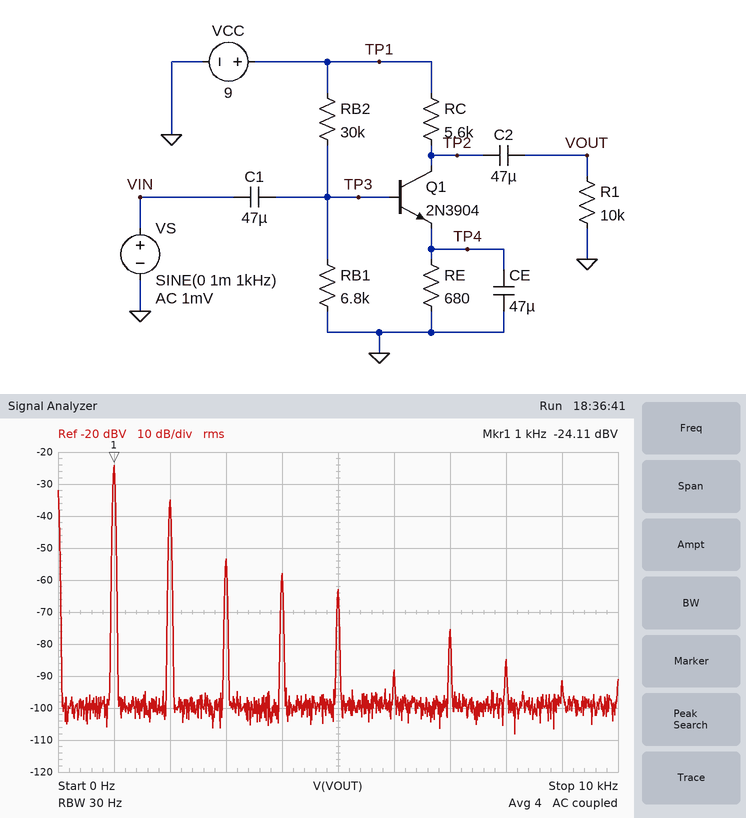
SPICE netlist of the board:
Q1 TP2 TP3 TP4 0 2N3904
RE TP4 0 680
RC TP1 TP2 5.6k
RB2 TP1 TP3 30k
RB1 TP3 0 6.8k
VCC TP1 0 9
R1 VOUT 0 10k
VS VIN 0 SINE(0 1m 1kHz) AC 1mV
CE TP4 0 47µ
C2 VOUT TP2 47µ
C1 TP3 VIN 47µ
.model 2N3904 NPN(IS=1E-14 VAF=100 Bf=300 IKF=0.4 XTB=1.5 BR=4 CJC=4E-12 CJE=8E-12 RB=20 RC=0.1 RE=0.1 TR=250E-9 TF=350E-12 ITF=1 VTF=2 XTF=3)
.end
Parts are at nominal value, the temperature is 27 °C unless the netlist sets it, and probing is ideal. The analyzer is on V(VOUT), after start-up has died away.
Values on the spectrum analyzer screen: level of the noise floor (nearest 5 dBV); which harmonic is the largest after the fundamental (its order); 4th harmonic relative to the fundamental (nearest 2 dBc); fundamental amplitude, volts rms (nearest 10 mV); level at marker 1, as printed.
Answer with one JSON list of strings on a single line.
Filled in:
["-100 dBV", "2", "-34 dBc", "60 mV", "-24.11 dBV"]
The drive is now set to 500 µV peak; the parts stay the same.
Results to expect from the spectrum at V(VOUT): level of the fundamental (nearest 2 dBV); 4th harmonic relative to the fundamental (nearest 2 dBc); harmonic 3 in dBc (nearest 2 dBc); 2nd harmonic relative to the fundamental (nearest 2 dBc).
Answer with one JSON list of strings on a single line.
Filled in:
["-30 dBV", "-52 dBc", "-32 dBc", "-14 dBc"]
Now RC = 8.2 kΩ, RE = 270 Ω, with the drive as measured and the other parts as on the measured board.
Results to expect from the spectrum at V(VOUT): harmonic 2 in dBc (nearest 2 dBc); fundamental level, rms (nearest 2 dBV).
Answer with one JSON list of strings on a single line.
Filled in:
["-32 dBc", "-60 dBV"]
